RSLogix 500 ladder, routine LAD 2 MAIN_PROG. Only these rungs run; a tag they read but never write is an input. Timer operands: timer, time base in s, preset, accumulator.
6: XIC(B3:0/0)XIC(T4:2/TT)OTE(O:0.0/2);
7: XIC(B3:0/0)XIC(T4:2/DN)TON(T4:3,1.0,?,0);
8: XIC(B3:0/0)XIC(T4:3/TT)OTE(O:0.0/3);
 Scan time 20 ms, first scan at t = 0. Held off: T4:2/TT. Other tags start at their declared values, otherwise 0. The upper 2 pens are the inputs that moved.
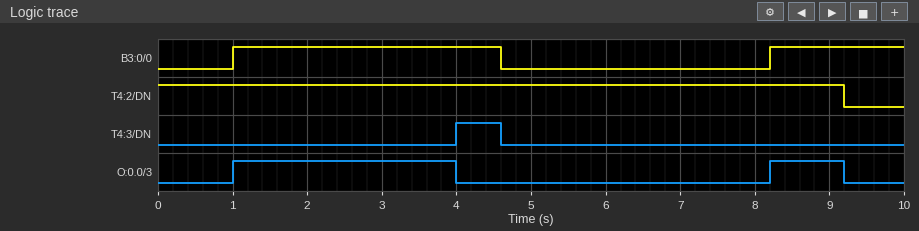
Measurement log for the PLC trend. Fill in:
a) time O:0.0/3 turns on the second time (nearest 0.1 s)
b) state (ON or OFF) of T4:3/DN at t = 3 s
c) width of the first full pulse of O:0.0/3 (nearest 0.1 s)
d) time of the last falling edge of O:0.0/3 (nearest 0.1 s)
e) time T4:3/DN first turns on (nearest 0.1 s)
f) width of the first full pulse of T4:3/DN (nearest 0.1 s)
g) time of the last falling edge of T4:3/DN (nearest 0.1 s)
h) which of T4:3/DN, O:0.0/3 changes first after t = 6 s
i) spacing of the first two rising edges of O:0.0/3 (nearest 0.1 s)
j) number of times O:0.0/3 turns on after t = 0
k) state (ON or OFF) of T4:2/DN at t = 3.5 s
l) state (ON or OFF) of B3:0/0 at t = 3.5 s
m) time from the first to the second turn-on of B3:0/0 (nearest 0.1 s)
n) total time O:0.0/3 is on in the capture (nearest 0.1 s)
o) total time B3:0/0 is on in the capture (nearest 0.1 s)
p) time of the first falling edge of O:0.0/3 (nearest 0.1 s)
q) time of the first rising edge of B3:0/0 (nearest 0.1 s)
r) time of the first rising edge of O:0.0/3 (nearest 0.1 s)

8.2 s
OFF
3.0 s
9.2 s
4.0 s
0.6 s
4.6 s
O:0.0/3
7.2 s
2
ON
ON
7.2 s
4.0 s
5.4 s
4.0 s
1.0 s
1.0 s
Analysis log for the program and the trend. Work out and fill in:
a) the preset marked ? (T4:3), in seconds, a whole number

3 s
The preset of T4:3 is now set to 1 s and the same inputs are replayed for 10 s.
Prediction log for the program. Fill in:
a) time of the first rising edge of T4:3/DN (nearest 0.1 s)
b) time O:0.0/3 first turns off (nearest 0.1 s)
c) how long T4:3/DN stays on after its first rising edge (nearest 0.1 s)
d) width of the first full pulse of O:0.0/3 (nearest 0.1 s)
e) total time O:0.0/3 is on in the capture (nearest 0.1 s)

2.0 s
2.0 s
2.6 s
1.0 s
2.0 s
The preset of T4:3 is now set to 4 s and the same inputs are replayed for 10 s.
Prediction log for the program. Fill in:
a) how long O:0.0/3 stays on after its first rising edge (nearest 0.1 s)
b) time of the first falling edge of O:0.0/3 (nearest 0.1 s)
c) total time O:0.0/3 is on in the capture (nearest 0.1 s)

3.6 s
4.6 s
4.6 s
